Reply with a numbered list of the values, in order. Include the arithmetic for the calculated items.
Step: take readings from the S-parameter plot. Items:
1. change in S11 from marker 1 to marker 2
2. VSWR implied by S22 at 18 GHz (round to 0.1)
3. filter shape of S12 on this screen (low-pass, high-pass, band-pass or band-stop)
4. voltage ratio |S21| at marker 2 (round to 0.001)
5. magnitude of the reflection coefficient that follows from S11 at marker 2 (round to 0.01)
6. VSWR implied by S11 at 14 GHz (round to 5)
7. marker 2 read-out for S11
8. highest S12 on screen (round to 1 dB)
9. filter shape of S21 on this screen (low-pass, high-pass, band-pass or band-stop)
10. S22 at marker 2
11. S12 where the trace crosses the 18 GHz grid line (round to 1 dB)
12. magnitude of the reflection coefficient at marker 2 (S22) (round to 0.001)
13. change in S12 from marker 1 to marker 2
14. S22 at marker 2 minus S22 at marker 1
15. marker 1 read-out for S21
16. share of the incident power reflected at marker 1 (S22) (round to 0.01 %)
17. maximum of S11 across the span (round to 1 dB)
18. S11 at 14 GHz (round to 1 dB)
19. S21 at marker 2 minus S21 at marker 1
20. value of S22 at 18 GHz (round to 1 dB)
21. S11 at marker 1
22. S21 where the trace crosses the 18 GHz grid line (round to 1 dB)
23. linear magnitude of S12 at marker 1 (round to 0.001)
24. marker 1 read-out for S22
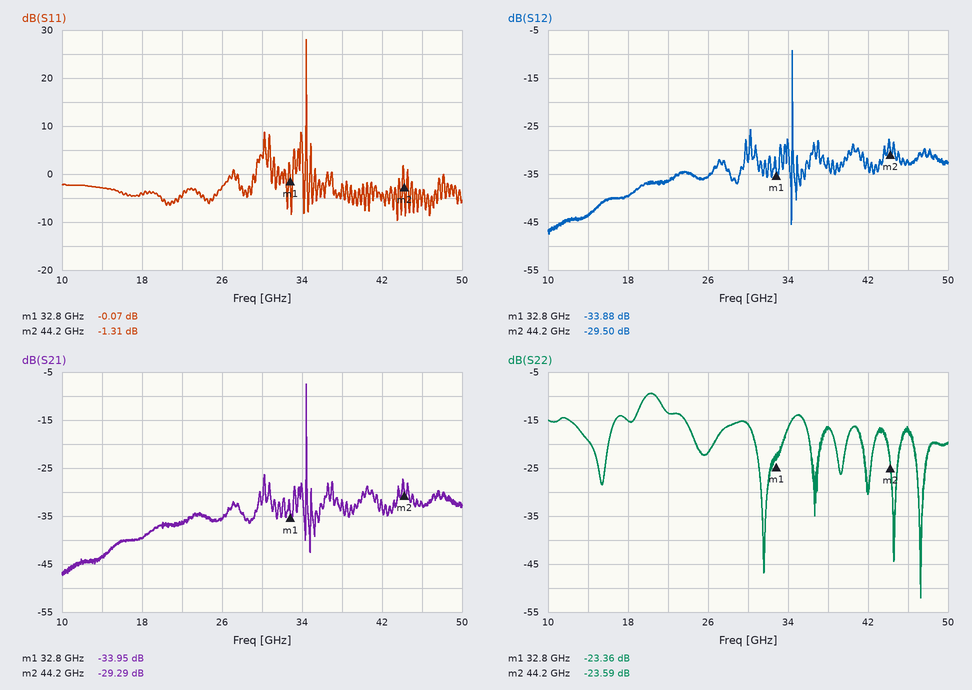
1. -1.31 − (-0.07) = -1.24 dB
2. |Γ| = 10^(-15/20) = 0.1778; VSWR = (1 + 0.1778)/(1 − 0.1778) ≈ 1.4
3. band-pass
4. 10^(-29.29/20) ≈ 0.034
5. 10^(-1.31/20) ≈ 0.86
6. |Γ| = 10^(-3/20) = 0.7079; VSWR = (1 + 0.7079)/(1 − 0.7079) ≈ 5.85, so 5 to the nearest 5
7. -1.31 dB
8. -9 dB
9. band-pass
10. -23.59 dB
11. -40 dB
12. 10^(-23.59/20) ≈ 0.066
13. -29.5 − (-33.88) = 4.38 dB
14. -23.59 − (-23.36) = -0.23 dB
15. -33.95 dB
16. 10^(-23.36/10) ≈ 0.46 %
17. 28 dB
18. -3 dB
19. -29.29 − (-33.95) = 4.66 dB
20. -15 dB
21. -0.07 dB
22. -40 dB
23. 10^(-33.88/20) ≈ 0.020
24. -23.36 dB
